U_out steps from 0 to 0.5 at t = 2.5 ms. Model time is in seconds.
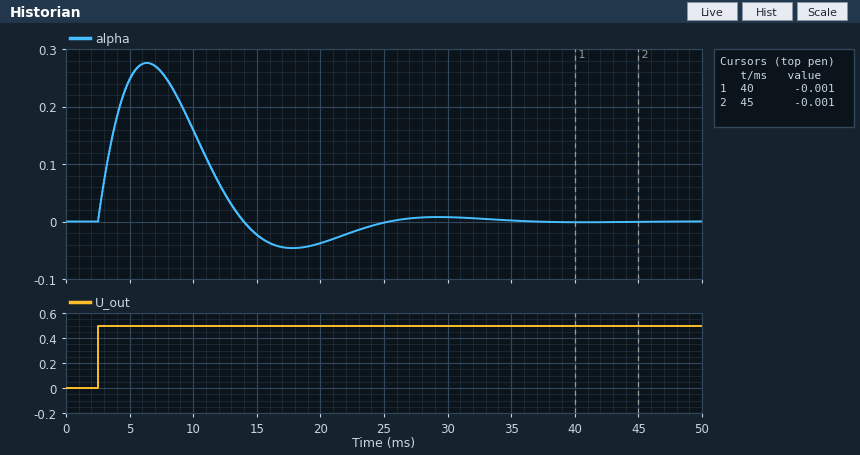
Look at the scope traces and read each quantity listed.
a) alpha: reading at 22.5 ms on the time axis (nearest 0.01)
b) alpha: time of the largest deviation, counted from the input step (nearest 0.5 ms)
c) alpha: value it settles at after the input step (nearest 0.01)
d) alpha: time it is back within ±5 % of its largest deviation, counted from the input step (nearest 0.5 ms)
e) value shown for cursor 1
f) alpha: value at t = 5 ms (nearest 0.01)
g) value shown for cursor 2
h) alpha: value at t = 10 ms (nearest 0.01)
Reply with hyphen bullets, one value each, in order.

- -0.02
- 4.0 ms
- 0.00
- 20.5 ms
- -0.001
- 0.25
- -0.001
- 0.16
